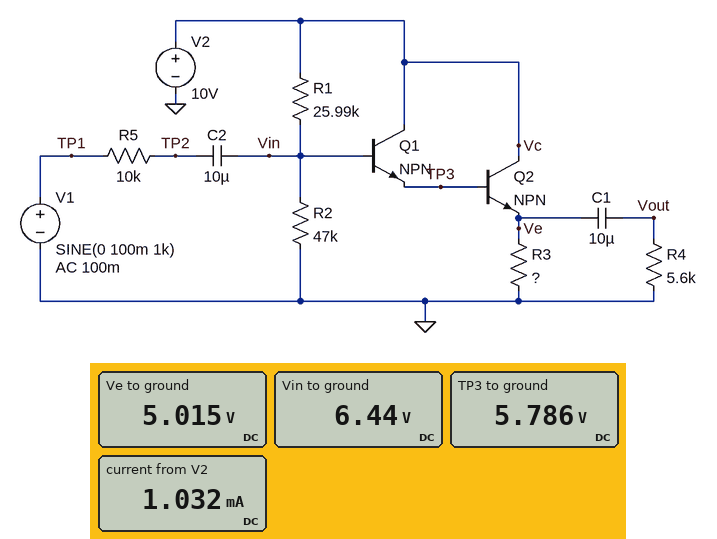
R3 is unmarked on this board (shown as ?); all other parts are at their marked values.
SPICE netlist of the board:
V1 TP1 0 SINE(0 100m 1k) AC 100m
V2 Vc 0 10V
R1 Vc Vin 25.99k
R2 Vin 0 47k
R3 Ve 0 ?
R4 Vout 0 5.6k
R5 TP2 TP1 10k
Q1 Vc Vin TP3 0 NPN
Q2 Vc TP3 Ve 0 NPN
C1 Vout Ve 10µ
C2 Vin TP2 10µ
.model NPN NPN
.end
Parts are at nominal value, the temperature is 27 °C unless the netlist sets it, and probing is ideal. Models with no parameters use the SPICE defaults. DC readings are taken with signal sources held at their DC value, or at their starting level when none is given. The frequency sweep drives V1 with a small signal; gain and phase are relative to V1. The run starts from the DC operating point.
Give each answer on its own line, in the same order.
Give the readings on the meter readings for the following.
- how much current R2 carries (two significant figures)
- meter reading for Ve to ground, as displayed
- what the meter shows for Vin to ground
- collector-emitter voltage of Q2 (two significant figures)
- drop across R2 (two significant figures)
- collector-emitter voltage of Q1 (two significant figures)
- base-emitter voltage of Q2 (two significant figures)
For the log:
140 µA
5.015 V
6.44 V
5.0 V
6.4 V
4.2 V
770 mV
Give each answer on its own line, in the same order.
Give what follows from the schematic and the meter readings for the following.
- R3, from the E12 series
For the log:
5.6 kΩ
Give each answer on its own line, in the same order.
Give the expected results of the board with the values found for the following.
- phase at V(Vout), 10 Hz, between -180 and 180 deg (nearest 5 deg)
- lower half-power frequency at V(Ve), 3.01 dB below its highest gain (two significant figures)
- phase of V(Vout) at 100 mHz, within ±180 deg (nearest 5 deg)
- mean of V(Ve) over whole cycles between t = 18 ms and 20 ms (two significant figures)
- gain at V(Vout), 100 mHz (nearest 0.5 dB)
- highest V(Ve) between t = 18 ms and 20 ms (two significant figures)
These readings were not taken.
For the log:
20 deg
580 mHz
170 deg
5.0 V
-49.0 dB
5.1 V
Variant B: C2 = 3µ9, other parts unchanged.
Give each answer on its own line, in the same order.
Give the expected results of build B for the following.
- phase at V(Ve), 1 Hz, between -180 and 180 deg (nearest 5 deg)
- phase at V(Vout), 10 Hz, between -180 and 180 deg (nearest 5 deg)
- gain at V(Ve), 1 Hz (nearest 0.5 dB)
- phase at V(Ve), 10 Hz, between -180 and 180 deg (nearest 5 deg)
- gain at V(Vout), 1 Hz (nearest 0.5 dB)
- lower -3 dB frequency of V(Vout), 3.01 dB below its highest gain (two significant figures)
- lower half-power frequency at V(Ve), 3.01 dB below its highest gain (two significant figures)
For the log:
55 deg
25 deg
-9.5 dB
10 deg
-19.0 dB
3.4 Hz
1.5 Hz
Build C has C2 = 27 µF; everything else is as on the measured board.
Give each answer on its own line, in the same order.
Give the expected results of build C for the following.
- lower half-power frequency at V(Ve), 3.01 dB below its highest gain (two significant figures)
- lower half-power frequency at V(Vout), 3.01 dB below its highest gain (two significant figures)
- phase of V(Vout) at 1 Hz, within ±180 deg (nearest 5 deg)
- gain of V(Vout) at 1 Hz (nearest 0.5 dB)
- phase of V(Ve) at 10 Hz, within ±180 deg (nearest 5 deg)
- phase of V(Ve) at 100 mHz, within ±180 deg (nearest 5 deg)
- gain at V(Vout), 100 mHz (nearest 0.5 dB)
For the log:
220 mHz
2.8 Hz
85 deg
-14.0 dB
0 deg
65 deg
-41.0 dB
